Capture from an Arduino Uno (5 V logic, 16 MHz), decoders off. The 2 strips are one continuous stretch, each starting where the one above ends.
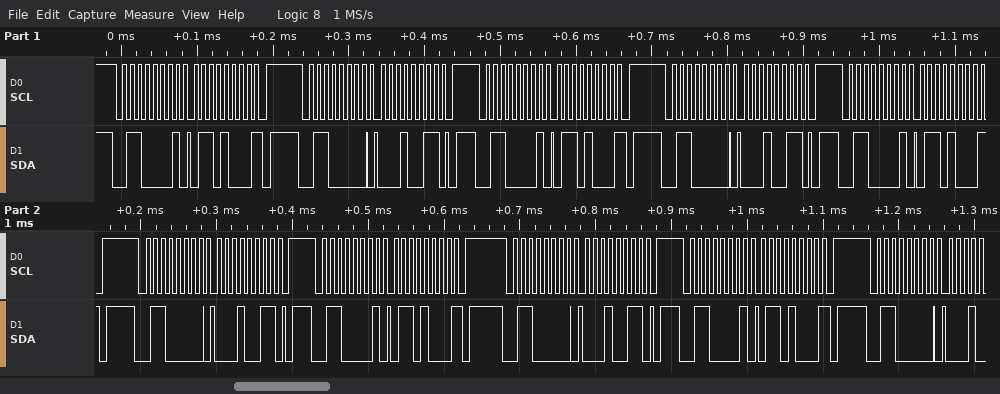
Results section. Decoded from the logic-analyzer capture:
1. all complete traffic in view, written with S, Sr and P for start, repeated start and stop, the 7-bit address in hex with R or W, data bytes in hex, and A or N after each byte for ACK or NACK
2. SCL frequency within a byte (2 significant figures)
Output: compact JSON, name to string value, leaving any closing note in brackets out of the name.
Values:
{"all complete traffic in view, written with S, Sr and P for start, repeated start and stop, the 7-bit address in hex with R or W, data bytes in hex, and A or N after each byte for ACK or NACK": "S 30R A 68 N P S 30W A 13 A P S 30R A 68 N P S 30W A 13 A P S 30R A 68 N P S 30W A 13 A P S 30R A 68 N P S 30W A 13 A P S 30R A 68 N P S 30W A", "SCL frequency within a byte": "100 kHz"}
